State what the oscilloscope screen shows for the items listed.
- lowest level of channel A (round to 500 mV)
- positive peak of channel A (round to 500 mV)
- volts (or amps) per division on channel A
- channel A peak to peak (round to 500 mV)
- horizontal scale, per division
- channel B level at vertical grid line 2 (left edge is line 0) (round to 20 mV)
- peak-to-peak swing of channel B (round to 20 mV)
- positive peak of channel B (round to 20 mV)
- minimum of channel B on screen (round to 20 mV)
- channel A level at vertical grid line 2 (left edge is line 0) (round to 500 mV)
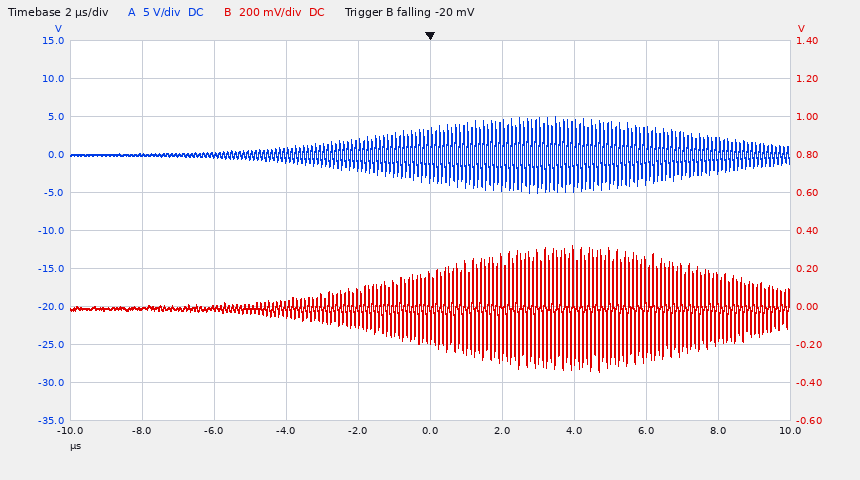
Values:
-5.0 V
5.0 V
5 V
10.0 V
2 µs
0 mV
660 mV
320 mV
-340 mV
0.0 V
